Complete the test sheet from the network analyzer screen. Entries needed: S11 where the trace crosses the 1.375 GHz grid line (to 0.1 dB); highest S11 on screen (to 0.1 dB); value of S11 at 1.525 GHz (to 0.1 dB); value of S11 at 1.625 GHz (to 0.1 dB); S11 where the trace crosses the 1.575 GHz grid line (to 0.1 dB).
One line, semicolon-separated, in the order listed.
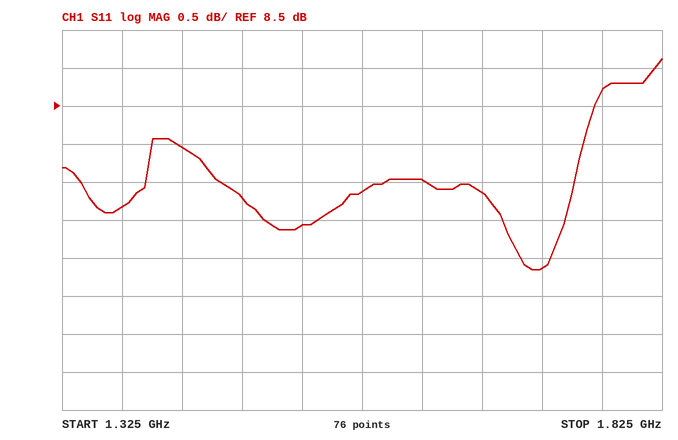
7.2 dB; 9.1 dB; 6.9 dB; 7.5 dB; 7.4 dB
